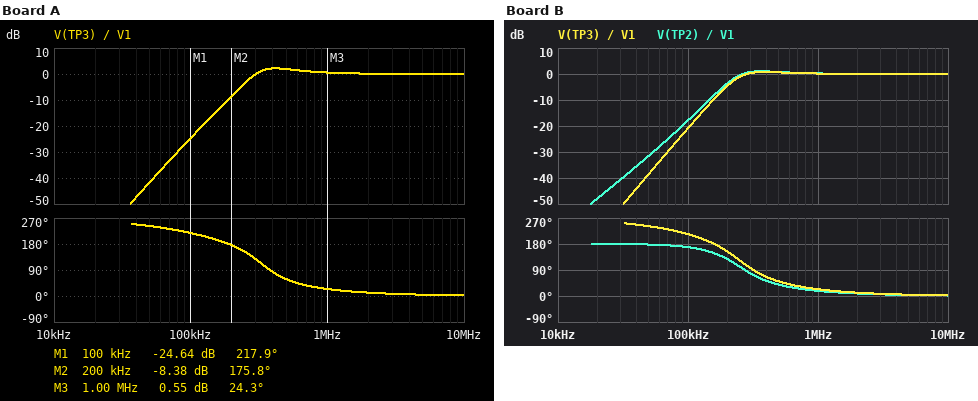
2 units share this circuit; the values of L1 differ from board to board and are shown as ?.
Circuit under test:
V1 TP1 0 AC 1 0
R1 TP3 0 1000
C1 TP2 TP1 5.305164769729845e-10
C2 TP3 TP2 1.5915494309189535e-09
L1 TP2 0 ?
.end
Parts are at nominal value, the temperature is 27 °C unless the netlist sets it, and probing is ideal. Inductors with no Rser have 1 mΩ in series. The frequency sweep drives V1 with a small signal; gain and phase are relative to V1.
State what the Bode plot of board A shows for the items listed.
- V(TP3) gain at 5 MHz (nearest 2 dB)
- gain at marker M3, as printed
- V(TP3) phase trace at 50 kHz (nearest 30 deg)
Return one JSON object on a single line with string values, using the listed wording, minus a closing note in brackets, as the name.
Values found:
{"V(TP3) gain at 5 MHz": "0 dB", "gain at marker M3, as printed": "0.55 dB", "V(TP3) phase trace at 50 kHz": "240 deg"}
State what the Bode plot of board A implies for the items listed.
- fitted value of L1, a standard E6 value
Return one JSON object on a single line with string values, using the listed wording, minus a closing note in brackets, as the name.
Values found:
{"fitted value of L1, a standard E6 value": "330 µH"}
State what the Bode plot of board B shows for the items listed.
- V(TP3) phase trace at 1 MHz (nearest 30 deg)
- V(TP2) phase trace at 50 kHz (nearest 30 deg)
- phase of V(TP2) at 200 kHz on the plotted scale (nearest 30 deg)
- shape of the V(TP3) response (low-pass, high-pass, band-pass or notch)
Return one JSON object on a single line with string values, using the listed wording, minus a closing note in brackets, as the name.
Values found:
{"V(TP3) phase trace at 1 MHz": "30 deg", "V(TP2) phase trace at 50 kHz": "180 deg", "phase of V(TP2) at 200 kHz on the plotted scale": "120 deg", "shape of the V(TP3) response": "high-pass"}
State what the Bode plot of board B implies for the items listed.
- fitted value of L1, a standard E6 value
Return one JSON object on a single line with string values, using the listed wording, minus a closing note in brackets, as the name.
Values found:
{"fitted value of L1, a standard E6 value": "470 µH"}
